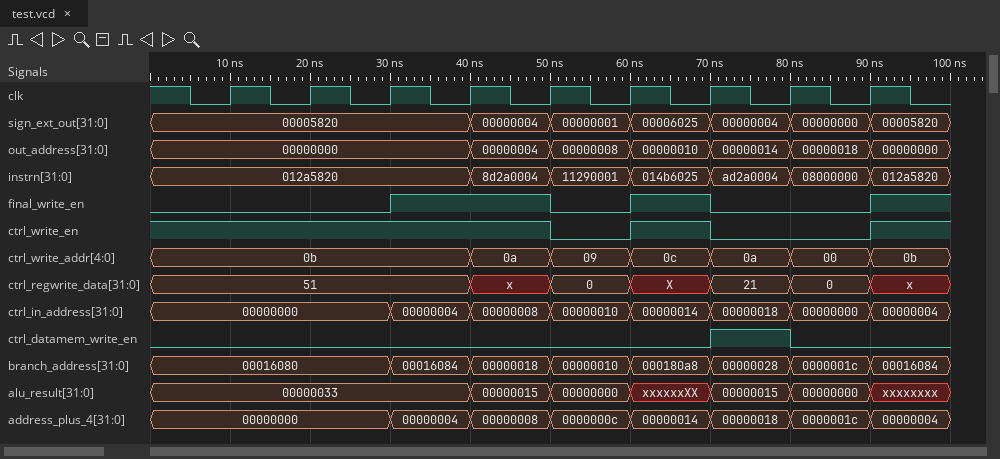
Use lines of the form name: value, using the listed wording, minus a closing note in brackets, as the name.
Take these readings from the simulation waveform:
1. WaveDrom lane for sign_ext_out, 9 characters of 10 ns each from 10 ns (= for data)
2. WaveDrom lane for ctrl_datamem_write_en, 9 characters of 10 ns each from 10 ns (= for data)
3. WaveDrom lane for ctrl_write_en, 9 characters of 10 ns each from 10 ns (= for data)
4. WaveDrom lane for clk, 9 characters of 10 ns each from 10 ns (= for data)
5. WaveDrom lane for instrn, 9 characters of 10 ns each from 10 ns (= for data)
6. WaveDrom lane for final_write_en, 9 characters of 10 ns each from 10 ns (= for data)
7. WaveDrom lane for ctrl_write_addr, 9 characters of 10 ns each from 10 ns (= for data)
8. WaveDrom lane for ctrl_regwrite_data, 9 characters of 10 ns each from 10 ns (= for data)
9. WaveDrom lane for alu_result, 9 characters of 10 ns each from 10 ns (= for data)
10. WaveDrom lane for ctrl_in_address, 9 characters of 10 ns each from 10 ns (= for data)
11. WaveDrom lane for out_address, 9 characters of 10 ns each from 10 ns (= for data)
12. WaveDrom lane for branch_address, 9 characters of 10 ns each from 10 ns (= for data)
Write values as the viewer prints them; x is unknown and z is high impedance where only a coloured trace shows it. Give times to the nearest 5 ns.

WaveDrom lane for sign_ext_out, 9 characters of 10 ns each from 10 ns: {name: 'sign_ext_out', wave: '=..======', data: '00005820 00000004 00000001 00006025 00000004 00000000 00005820'}
WaveDrom lane for ctrl_datamem_write_en, 9 characters of 10 ns each from 10 ns: {name: 'ctrl_datamem_write_en', wave: '0.....10.'}
WaveDrom lane for ctrl_write_en, 9 characters of 10 ns each from 10 ns: {name: 'ctrl_write_en', wave: '1...010.1'}
WaveDrom lane for clk, 9 characters of 10 ns each from 10 ns: {name: 'clk', wave: 'p........'}
WaveDrom lane for instrn, 9 characters of 10 ns each from 10 ns: {name: 'instrn', wave: '=..======', data: '012a5820 8d2a0004 11290001 014b6025 ad2a0004 08000000 012a5820'}
WaveDrom lane for final_write_en, 9 characters of 10 ns each from 10 ns: {name: 'final_write_en', wave: '0.1.010.1'}
WaveDrom lane for ctrl_write_addr, 9 characters of 10 ns each from 10 ns: {name: 'ctrl_write_addr', wave: '=..======', data: '0b 0a 09 0c 0a 00 0b'}
WaveDrom lane for ctrl_regwrite_data, 9 characters of 10 ns each from 10 ns: {name: 'ctrl_regwrite_data', wave: '=..x====x', data: '51 0 X 21 0'}
WaveDrom lane for alu_result, 9 characters of 10 ns each from 10 ns: {name: 'alu_result', wave: '=..=====x', data: '00000033 00000015 00000000 xxxxxxXX 00000015 00000000'}
WaveDrom lane for ctrl_in_address, 9 characters of 10 ns each from 10 ns: {name: 'ctrl_in_address', wave: '=.=======', data: '00000000 00000004 00000008 00000010 00000014 00000018 00000000 00000004'}
WaveDrom lane for out_address, 9 characters of 10 ns each from 10 ns: {name: 'out_address', wave: '=..======', data: '00000000 00000004 00000008 00000010 00000014 00000018 00000000'}
WaveDrom lane for branch_address, 9 characters of 10 ns each from 10 ns: {name: 'branch_address', wave: '=.=======', data: '00016080 00016084 00000018 00000010 000180a8 00000028 0000001c 00016084'}
